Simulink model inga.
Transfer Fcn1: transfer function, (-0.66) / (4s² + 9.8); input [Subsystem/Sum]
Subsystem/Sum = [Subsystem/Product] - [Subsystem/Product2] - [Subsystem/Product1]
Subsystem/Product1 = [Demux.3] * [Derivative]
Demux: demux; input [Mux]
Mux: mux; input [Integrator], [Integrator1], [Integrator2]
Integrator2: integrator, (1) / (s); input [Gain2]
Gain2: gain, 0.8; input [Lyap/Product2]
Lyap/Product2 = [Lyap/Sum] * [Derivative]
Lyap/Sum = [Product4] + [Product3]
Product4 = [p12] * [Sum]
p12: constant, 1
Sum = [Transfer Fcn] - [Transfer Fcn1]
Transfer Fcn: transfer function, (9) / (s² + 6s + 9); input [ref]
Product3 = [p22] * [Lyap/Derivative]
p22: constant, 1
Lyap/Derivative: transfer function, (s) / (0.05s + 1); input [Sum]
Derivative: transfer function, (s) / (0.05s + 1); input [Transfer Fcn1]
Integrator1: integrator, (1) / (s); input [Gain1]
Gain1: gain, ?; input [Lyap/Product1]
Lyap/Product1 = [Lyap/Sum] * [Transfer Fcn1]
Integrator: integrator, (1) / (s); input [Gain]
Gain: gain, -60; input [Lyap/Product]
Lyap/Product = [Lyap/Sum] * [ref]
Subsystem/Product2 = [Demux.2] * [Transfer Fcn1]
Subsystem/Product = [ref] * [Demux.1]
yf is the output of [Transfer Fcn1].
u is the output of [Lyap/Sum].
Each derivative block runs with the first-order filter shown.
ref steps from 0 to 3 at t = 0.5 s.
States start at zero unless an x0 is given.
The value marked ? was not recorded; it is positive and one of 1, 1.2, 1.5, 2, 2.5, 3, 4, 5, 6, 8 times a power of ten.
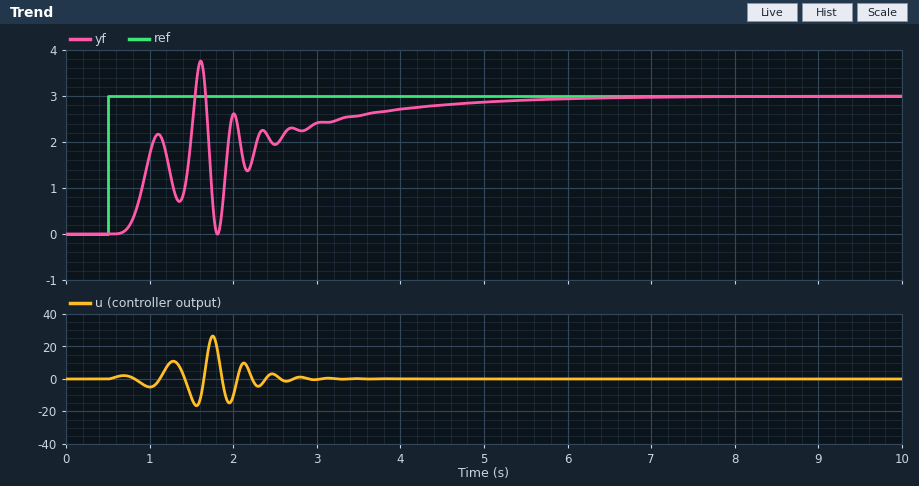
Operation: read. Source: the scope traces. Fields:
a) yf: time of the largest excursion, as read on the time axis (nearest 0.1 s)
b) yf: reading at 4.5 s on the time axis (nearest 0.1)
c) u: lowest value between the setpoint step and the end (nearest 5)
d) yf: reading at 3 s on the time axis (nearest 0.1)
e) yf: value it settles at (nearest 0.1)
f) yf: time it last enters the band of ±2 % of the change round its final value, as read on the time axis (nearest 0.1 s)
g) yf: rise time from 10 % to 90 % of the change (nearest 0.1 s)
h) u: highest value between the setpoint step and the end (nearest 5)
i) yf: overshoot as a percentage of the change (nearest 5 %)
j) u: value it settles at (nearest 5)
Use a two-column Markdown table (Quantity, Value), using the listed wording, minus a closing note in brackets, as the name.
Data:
| Quantity | Value |
|---|---|
| yf: time of the largest excursion, as read on the time axis | 1.6 s |
| yf: reading at 4.5 s on the time axis | 2.8 |
| u: lowest value between the setpoint step and the end | -15 |
| yf: reading at 3 s on the time axis | 2.4 |
| yf: value it settles at | 3.0 |
| yf: time it last enters the band of ±2 % of the change round its final value, as read on the time axis | 6.0 s |
| yf: rise time from 10 % to 90 % of the change | 0.7 s |
| u: highest value between the setpoint step and the end | 25 |
| yf: overshoot as a percentage of the change | 25 % |
| u: value it settles at | 0 |
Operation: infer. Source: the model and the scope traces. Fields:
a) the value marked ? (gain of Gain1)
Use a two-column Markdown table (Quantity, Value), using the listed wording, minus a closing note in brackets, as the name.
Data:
| Quantity | Value |
|---|---|
| the value marked ? | 100 |
